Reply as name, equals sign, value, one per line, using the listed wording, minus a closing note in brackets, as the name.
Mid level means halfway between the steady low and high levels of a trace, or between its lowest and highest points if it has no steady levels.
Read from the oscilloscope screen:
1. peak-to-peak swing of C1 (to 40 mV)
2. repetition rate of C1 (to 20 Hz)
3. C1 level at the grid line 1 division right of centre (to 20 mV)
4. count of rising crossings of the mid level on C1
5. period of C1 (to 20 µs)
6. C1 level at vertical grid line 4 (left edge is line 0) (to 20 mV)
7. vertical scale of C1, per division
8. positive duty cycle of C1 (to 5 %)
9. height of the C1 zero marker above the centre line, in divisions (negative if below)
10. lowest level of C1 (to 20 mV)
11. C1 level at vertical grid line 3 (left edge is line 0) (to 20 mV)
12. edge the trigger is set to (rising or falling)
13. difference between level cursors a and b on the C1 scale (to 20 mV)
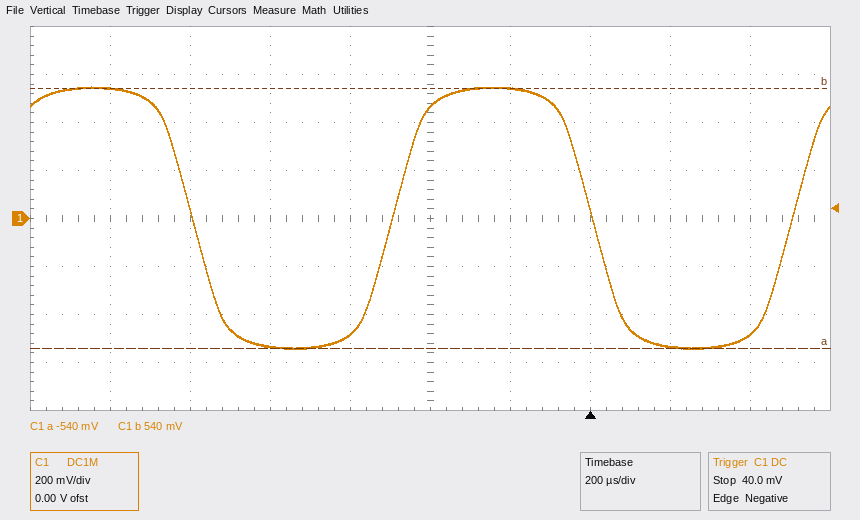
peak-to-peak swing of C1 = 1.08 V
repetition rate of C1 = 1.00 kHz
C1 level at the grid line 1 division right of centre = 540 mV
count of rising crossings of the mid level on C1 = 2
period of C1 = 1.00 ms
C1 level at vertical grid line 4 (left edge is line 0) = -480 mV
vertical scale of C1, per division = 200 mV
positive duty cycle of C1 = 50 %
height of the C1 zero marker above the centre line, in divisions = 0.0 div
lowest level of C1 = -540 mV
C1 level at vertical grid line 3 (left edge is line 0) = -540 mV
edge the trigger is set to = falling
difference between level cursors a and b on the C1 scale = 1.08 V
